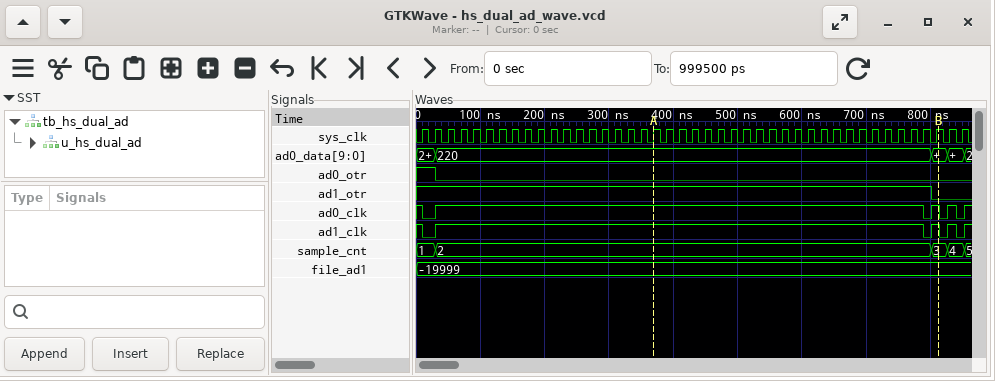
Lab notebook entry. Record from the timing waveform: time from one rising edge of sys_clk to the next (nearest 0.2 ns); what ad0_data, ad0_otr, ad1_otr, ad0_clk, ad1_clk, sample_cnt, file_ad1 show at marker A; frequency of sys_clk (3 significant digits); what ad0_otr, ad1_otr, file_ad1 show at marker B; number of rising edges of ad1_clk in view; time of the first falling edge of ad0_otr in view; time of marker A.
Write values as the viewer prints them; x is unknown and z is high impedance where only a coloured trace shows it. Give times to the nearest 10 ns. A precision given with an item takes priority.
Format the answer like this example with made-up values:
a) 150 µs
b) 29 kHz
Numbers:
a) 20 ns
b) ad0_data=220, ad0_otr=0, ad1_otr=1, ad0_clk=1, ad1_clk=1, sample_cnt=2, file_ad1=-19999
c) 50.0 MHz
d) ad0_otr=0, ad1_otr=0, file_ad1=-19999
e) 4
f) 30 ns
g) 370 ns
